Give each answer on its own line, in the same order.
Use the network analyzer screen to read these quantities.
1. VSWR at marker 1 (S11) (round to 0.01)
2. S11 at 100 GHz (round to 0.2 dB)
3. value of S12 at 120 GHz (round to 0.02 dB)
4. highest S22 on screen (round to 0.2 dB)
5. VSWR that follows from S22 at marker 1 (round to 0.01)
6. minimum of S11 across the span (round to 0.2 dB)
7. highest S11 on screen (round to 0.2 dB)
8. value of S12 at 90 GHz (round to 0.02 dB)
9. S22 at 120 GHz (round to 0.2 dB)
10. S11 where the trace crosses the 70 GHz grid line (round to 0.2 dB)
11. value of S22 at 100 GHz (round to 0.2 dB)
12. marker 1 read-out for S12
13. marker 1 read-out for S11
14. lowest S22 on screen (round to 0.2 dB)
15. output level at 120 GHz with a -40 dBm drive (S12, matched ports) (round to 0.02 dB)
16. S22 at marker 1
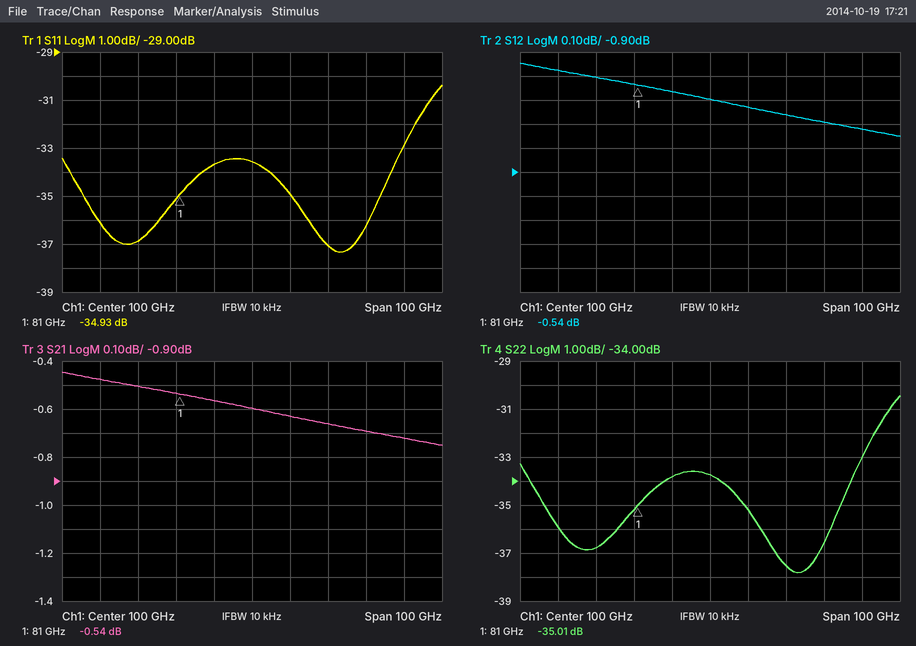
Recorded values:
1.04
-33.6 dB
-0.66 dB
-30.4 dB
1.04
-37.4 dB
-30.4 dB
-0.56 dB
-37.6 dB
-36.8 dB
-33.8 dB
-0.54 dB
-34.93 dB
-37.8 dB
-40.66 dBm
-35.01 dB
